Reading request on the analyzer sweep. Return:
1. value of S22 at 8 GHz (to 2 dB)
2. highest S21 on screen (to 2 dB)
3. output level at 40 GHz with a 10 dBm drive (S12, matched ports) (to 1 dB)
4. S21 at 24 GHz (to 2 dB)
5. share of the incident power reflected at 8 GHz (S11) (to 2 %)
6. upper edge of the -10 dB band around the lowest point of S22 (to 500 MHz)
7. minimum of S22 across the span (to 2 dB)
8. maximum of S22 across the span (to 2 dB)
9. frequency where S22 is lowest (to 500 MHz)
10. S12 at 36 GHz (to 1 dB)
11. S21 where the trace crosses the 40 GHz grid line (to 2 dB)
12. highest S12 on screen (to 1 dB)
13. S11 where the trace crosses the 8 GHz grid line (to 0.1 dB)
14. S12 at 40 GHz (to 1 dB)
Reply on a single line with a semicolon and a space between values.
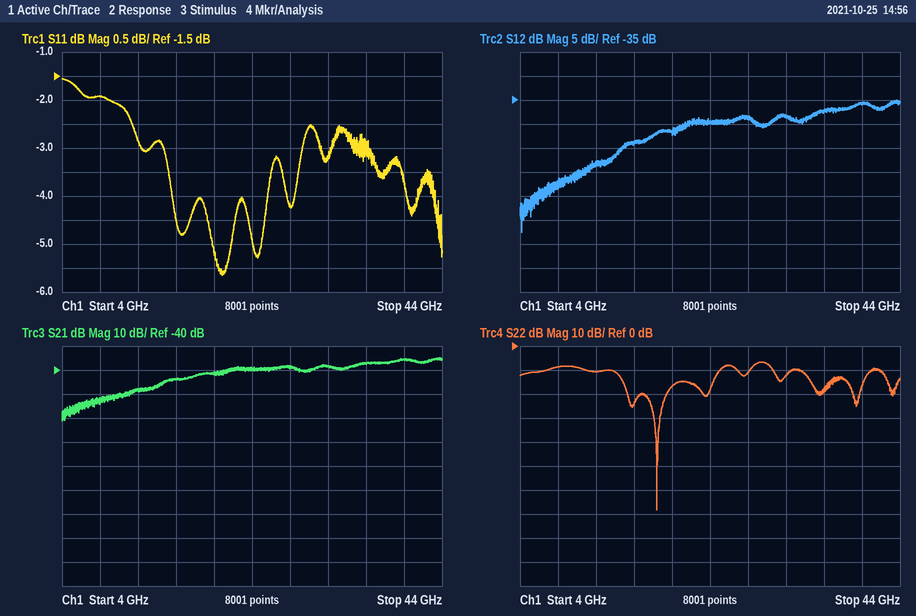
-8 dB; -34 dB; -26 dBm; -40 dB; 64 %; 25.0 GHz; -68 dB; -6 dB; 18.5 GHz; -37 dB; -36 dB; -35 dB; -1.9 dB; -36 dB
